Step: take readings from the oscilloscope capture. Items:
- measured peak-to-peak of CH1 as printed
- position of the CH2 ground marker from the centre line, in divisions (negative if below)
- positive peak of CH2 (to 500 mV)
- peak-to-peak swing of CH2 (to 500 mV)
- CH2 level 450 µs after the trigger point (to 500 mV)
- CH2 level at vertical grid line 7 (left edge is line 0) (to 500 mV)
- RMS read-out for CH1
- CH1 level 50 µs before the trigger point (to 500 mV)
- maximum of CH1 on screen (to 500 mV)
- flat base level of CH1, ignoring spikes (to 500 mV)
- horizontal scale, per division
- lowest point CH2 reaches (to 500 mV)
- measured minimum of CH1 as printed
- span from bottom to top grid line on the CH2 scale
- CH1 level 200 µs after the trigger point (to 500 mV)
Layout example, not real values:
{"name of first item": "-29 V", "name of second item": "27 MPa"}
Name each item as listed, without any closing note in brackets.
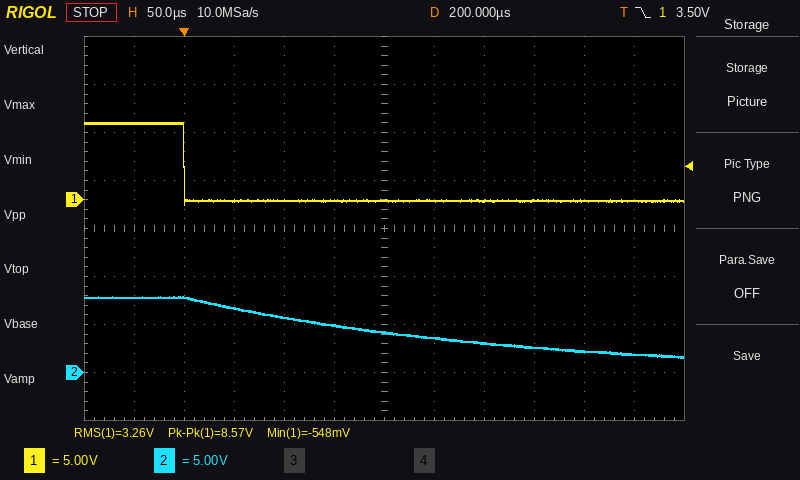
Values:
{"measured peak-to-peak of CH1 as printed": "8.57 V", "position of the CH2 ground marker from the centre line, in divisions": "-3.0 div", "positive peak of CH2": "8.0 V", "peak-to-peak swing of CH2": "6.5 V", "CH2 level 450 µs after the trigger point": "2.0 V", "CH2 level at vertical grid line 7 (left edge is line 0)": "3.5 V", "RMS read-out for CH1": "3.26 V", "CH1 level 50 µs before the trigger point": "8.0 V", "maximum of CH1 on screen": "8.0 V", "flat base level of CH1, ignoring spikes": "0.0 V", "horizontal scale, per division": "50 µs", "lowest point CH2 reaches": "1.5 V", "measured minimum of CH1 as printed": "-548 mV", "span from bottom to top grid line on the CH2 scale": "40 V", "CH1 level 200 µs after the trigger point": "0.0 V"}
